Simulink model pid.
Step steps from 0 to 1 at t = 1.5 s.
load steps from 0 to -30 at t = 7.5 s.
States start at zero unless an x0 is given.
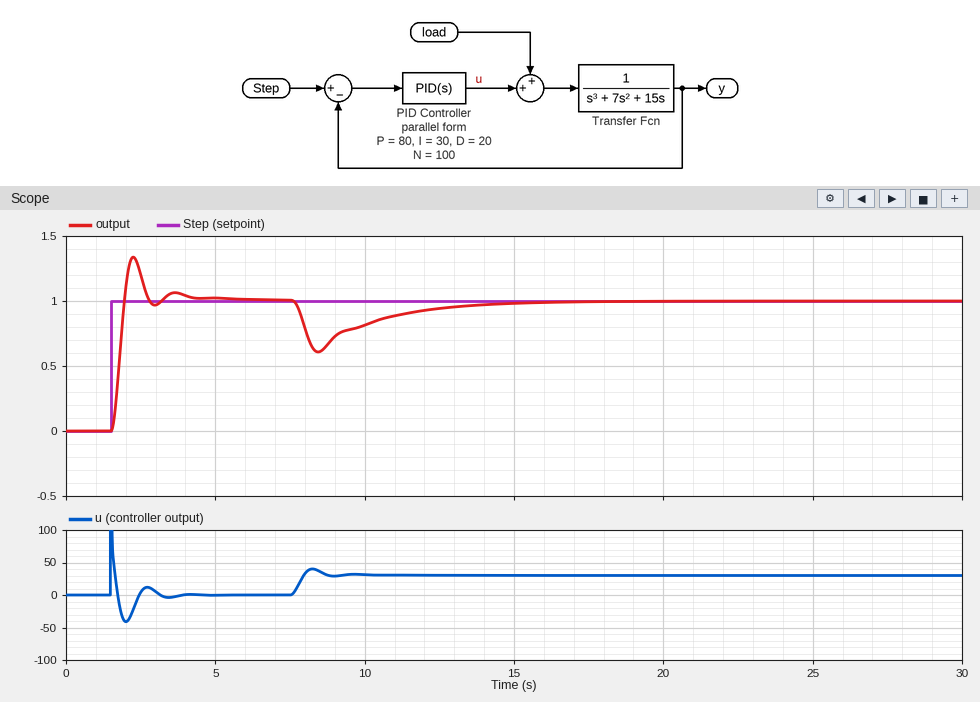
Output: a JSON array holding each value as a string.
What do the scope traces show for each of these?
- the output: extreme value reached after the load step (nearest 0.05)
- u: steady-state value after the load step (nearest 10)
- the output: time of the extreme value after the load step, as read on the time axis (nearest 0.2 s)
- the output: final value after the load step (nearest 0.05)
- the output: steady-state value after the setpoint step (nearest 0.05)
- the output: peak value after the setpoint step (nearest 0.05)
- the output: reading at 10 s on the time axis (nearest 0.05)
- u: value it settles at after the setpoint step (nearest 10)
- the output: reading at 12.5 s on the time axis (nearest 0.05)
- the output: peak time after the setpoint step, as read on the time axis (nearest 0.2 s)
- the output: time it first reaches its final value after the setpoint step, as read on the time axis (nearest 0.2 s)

["0.60", "30", "8.4 s", "1.00", "1.00", "1.35", "0.80", "0", "0.95", "2.2 s", "2.0 s"]
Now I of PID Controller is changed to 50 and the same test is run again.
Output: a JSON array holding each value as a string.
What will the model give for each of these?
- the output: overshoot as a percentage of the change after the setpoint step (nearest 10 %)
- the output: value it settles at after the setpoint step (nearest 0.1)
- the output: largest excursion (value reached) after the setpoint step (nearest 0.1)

["40 %", "1.0", "1.4"]
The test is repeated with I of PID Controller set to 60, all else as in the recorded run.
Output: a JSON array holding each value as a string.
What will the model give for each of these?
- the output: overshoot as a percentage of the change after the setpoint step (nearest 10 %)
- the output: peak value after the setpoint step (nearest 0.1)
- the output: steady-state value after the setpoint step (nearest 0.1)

["40 %", "1.4", "1.0"]
